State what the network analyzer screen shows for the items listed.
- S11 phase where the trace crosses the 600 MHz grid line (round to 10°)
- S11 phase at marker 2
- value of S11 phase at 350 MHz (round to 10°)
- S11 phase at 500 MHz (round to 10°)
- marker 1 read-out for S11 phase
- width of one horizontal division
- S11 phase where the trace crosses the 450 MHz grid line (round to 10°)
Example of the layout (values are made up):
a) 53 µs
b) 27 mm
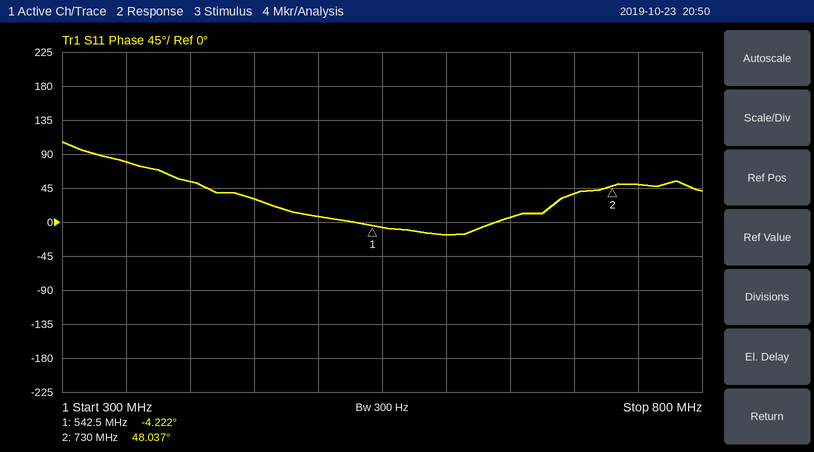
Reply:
a) -20°
b) 48.037°
c) 80°
d) 10°
e) -4.222°
f) 50 MHz
g) 30°
